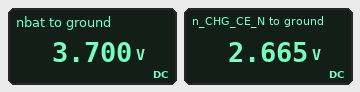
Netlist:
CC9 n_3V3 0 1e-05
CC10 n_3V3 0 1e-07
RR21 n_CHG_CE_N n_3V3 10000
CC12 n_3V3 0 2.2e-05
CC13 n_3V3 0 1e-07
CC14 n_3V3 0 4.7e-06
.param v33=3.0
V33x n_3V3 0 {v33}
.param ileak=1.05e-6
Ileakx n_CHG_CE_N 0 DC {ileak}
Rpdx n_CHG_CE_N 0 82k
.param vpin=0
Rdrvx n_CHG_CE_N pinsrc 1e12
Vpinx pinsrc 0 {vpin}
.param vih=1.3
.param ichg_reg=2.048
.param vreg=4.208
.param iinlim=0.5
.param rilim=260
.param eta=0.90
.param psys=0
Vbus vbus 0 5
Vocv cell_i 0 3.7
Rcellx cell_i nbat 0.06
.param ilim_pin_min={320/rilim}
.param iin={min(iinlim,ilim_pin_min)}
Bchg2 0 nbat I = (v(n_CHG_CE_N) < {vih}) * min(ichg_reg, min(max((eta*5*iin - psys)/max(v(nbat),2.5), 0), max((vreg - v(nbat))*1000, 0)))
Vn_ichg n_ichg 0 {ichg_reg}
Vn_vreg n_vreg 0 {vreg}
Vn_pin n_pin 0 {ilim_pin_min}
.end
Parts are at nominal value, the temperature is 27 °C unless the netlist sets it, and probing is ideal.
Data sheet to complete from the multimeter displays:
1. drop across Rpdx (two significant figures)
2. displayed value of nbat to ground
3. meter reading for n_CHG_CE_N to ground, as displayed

2.7 V
3.700 V
2.665 V
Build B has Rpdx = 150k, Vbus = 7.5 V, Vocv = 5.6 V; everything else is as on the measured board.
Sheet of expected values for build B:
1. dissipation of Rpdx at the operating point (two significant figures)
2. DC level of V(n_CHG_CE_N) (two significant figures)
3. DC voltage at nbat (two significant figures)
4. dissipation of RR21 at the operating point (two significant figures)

52 µW
2.8 V
5.6 V
3.9 µW
